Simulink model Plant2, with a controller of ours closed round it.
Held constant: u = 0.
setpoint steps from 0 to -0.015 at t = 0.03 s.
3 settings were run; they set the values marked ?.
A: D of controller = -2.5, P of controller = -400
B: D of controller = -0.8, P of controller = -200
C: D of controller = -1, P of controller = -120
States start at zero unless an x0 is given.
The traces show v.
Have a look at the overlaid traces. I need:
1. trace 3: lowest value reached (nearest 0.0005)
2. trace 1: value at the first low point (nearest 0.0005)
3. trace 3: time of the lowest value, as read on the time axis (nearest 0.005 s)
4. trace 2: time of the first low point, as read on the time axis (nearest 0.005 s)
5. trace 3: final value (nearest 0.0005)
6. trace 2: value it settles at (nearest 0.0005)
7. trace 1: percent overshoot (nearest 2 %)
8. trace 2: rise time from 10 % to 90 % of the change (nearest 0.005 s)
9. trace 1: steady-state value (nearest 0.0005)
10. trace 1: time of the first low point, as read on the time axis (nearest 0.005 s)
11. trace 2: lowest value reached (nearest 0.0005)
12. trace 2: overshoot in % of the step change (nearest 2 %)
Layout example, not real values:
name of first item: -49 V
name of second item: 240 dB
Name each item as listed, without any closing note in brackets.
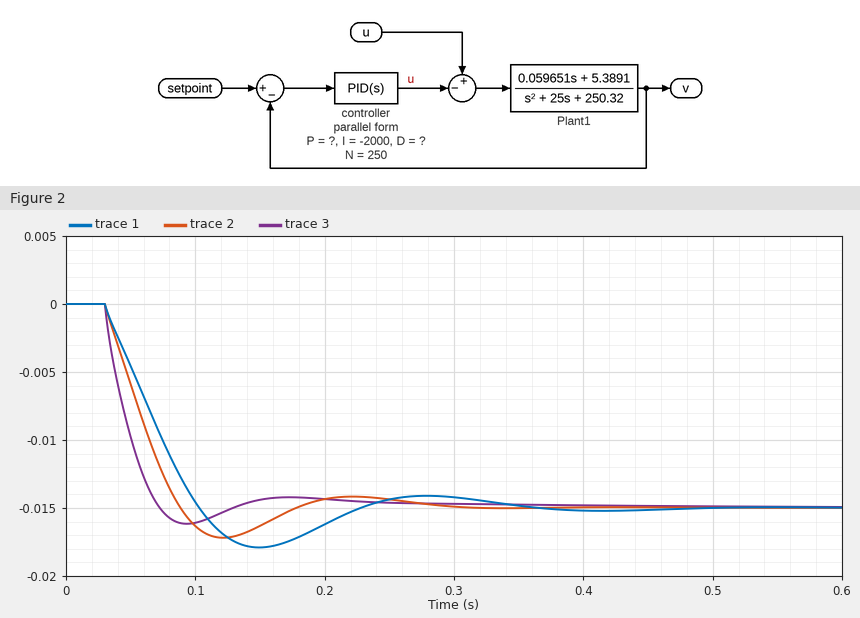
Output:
trace 3: lowest value reached: -0.0160
trace 1: value at the first low point: -0.0180
trace 3: time of the lowest value, as read on the time axis: 0.095 s
trace 2: time of the first low point, as read on the time axis: 0.120 s
trace 3: final value: -0.0150
trace 2: value it settles at: -0.0150
trace 1: percent overshoot: 20 %
trace 2: rise time from 10 % to 90 % of the change: 0.045 s
trace 1: steady-state value: -0.0150
trace 1: time of the first low point, as read on the time axis: 0.150 s
trace 2: lowest value reached: -0.0170
trace 2: overshoot in % of the step change: 14 %
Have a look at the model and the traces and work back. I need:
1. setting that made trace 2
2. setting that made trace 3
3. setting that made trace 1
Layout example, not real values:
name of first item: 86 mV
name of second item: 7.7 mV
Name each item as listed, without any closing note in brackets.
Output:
setting that made trace 2: B
setting that made trace 3: A
setting that made trace 1: C
